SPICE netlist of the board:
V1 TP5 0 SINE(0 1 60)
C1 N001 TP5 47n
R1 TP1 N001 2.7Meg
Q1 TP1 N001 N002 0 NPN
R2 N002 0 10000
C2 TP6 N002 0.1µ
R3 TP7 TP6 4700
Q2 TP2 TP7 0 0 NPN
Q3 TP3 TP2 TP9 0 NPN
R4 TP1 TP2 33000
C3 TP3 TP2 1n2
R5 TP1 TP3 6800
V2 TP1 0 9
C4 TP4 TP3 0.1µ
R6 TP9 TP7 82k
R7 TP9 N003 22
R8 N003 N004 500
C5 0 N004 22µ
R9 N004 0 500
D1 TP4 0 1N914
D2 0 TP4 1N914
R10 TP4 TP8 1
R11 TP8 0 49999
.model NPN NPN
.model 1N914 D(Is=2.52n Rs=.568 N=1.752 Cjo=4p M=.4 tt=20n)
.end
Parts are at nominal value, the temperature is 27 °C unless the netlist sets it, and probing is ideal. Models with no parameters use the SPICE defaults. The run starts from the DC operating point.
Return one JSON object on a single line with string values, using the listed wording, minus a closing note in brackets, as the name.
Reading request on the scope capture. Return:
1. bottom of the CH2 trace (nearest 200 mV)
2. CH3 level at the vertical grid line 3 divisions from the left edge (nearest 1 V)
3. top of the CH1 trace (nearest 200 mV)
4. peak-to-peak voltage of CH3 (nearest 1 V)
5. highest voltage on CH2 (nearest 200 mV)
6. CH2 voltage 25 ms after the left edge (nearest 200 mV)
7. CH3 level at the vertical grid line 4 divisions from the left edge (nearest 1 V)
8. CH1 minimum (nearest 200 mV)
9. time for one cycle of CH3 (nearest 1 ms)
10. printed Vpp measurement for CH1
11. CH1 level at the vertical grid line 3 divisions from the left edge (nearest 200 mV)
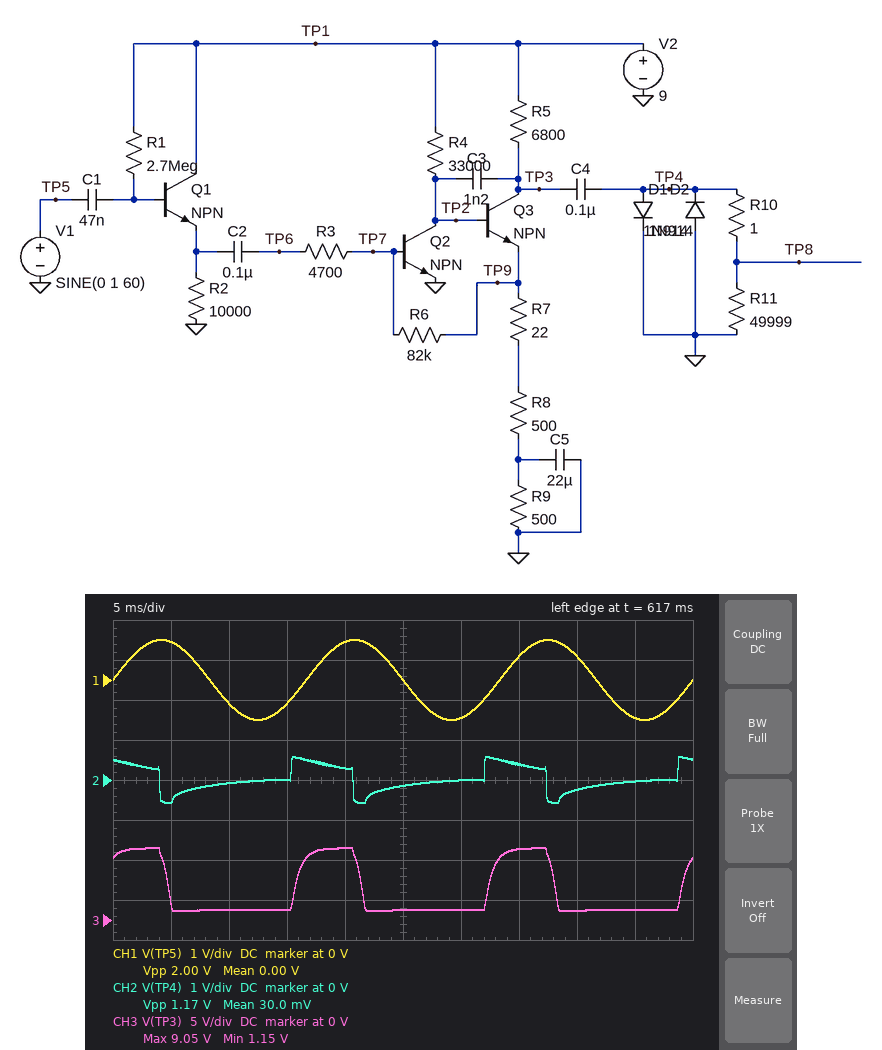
{"bottom of the CH2 trace": "-600 mV", "CH3 level at the vertical grid line 3 divisions from the left edge": "1 V", "top of the CH1 trace": "1.0 V", "peak-to-peak voltage of CH3": "8 V", "highest voltage on CH2": "600 mV", "CH2 voltage 25 ms after the left edge": "-200 mV", "CH3 level at the vertical grid line 4 divisions from the left edge": "9 V", "CH1 minimum": "-1.0 V", "time for one cycle of CH3": "17 ms", "printed Vpp measurement for CH1": "2.00 V", "CH1 level at the vertical grid line 3 divisions from the left edge": "-600 mV"}
